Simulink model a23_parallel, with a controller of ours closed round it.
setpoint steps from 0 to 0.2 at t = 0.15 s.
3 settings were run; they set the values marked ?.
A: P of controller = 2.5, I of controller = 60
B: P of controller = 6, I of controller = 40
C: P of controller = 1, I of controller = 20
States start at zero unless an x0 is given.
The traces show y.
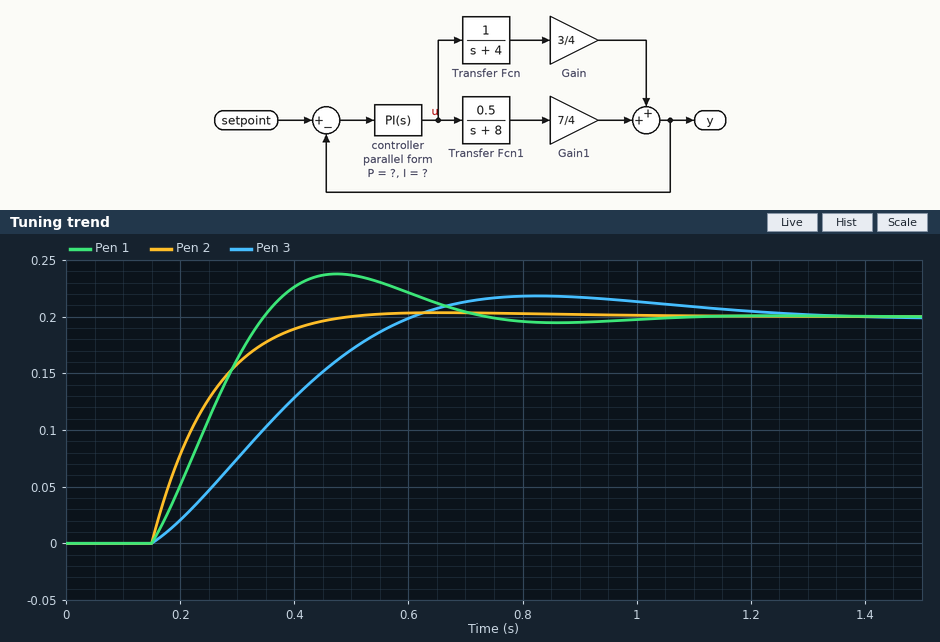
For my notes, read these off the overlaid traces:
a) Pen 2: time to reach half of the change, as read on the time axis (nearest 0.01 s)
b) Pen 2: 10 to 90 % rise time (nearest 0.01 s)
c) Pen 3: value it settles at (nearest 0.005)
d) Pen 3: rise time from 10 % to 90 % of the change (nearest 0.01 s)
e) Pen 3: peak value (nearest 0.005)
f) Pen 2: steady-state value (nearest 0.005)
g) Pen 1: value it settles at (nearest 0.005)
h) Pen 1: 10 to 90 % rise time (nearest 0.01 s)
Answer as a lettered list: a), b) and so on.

a) 0.22 s
b) 0.20 s
c) 0.200
d) 0.33 s
e) 0.220
f) 0.200
g) 0.200
h) 0.15 s
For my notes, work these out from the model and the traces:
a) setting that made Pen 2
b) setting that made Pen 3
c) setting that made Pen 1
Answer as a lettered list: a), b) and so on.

a) B
b) C
c) A
